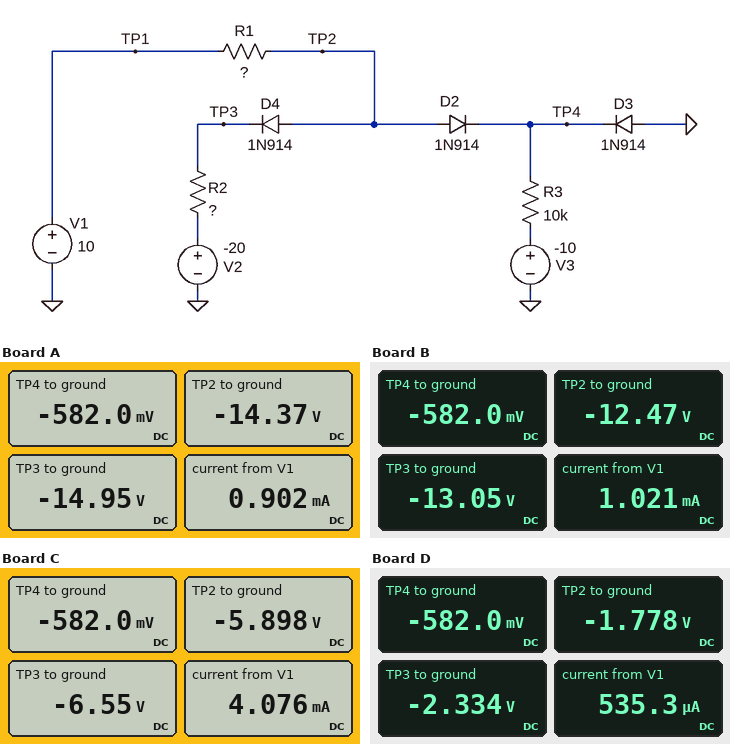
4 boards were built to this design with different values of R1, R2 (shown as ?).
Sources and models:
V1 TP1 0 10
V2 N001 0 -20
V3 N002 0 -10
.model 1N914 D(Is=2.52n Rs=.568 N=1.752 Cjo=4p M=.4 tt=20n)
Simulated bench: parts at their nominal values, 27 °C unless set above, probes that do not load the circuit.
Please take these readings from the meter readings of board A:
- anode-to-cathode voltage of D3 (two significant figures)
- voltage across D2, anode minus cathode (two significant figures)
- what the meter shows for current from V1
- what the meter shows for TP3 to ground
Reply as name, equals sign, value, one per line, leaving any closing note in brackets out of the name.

anode-to-cathode voltage of D3 = 580 mV
voltage across D2, anode minus cathode = -14 V
what the meter shows for current from V1 = 0.902 mA
what the meter shows for TP3 to ground = -14.95 V
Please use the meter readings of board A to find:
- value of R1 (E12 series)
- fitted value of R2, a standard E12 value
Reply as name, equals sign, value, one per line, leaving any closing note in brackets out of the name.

value of R1 = 27 kΩ
fitted value of R2, a standard E12 value = 5.6 kΩ
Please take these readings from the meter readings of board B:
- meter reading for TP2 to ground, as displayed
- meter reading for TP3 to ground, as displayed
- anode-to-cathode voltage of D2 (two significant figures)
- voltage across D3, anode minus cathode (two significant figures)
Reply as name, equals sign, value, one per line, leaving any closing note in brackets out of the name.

meter reading for TP2 to ground, as displayed = -12.47 V
meter reading for TP3 to ground, as displayed = -13.05 V
anode-to-cathode voltage of D2 = -12 V
voltage across D3, anode minus cathode = 580 mV
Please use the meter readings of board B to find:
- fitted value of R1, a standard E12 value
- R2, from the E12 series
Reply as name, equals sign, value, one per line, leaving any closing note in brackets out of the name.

fitted value of R1, a standard E12 value = 22 kΩ
R2, from the E12 series = 6.8 kΩ
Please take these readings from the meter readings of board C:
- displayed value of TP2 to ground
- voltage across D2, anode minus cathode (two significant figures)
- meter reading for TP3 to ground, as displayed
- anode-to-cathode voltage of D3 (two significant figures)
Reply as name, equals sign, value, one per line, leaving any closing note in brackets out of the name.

displayed value of TP2 to ground = -5.898 V
voltage across D2, anode minus cathode = -5.3 V
meter reading for TP3 to ground, as displayed = -6.55 V
anode-to-cathode voltage of D3 = 580 mV
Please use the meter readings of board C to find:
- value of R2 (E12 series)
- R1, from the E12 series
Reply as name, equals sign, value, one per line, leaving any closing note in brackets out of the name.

value of R2 = 3.3 kΩ
R1, from the E12 series = 3.9 kΩ
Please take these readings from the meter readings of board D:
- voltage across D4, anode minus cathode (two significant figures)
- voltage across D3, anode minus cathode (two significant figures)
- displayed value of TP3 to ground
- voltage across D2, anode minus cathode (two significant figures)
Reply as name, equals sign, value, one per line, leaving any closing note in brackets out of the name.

voltage across D4, anode minus cathode = 560 mV
voltage across D3, anode minus cathode = 580 mV
displayed value of TP3 to ground = -2.334 V
voltage across D2, anode minus cathode = -1.2 V
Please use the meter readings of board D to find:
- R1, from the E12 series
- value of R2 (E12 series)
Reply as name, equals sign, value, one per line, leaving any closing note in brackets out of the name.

R1, from the E12 series = 22 kΩ
value of R2 = 33 kΩ
